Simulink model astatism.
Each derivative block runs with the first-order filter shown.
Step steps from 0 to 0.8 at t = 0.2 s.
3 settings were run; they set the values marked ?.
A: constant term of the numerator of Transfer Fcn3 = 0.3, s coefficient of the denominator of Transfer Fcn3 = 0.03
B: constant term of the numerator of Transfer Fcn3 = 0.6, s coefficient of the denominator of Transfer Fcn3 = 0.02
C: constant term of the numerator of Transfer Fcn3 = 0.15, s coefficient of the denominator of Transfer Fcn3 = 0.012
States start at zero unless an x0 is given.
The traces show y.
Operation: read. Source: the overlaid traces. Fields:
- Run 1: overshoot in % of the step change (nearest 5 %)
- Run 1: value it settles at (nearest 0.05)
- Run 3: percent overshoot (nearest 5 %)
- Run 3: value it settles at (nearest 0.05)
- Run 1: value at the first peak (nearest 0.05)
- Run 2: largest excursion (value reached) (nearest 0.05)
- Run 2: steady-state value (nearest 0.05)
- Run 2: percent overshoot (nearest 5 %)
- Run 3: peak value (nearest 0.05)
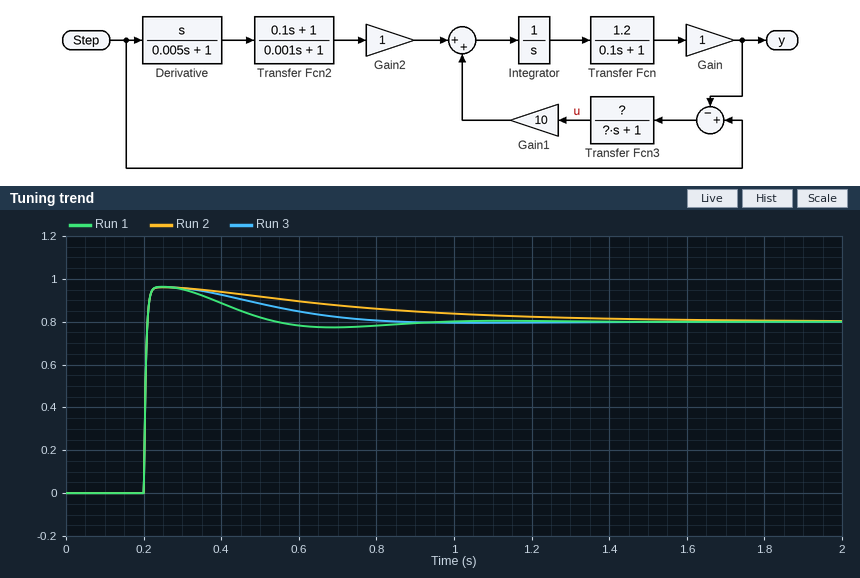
20 %
0.80
20 %
0.80
0.95
0.95
0.80
20 %
0.95
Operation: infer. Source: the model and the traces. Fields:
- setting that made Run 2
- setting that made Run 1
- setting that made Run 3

C
B
A
